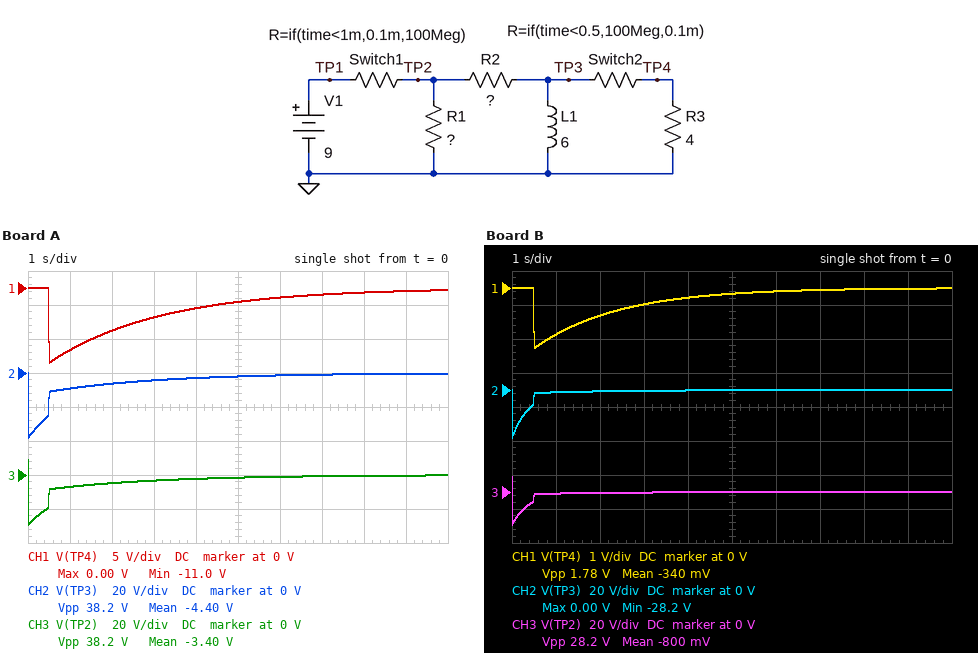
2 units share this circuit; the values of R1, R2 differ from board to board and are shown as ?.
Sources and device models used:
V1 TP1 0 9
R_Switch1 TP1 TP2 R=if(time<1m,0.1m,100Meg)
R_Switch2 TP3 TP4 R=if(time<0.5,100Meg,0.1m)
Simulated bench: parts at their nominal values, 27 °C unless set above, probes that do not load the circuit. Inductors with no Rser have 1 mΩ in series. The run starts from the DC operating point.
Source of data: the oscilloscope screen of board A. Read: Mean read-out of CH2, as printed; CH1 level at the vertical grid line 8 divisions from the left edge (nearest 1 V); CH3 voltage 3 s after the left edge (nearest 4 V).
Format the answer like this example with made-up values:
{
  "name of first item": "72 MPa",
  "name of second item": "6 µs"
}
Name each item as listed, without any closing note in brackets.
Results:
{
  "Mean read-out of CH2, as printed": "-4.40 V",
  "CH1 level at the vertical grid line 8 divisions from the left edge": "-1 V",
  "CH3 voltage 3 s after the left edge": "-4 V"
}
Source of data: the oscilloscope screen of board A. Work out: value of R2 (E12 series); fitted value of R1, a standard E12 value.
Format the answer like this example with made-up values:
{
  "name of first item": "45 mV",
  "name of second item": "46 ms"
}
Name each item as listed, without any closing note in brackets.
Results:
{
  "value of R2": "1.2 Ω",
  "fitted value of R1, a standard E12 value": "3.9 Ω"
}
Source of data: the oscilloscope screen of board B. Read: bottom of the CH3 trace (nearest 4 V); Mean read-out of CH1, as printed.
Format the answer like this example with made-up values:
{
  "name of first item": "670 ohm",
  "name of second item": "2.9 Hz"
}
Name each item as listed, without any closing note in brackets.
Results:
{
  "bottom of the CH3 trace": "-20 V",
  "Mean read-out of CH1, as printed": "-340 mV"
}
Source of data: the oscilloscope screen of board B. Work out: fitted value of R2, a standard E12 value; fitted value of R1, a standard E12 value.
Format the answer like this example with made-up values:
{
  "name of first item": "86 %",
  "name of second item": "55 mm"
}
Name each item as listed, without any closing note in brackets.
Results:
{
  "fitted value of R2, a standard E12 value": "4.7 Ω",
  "fitted value of R1, a standard E12 value": "10 Ω"
}
